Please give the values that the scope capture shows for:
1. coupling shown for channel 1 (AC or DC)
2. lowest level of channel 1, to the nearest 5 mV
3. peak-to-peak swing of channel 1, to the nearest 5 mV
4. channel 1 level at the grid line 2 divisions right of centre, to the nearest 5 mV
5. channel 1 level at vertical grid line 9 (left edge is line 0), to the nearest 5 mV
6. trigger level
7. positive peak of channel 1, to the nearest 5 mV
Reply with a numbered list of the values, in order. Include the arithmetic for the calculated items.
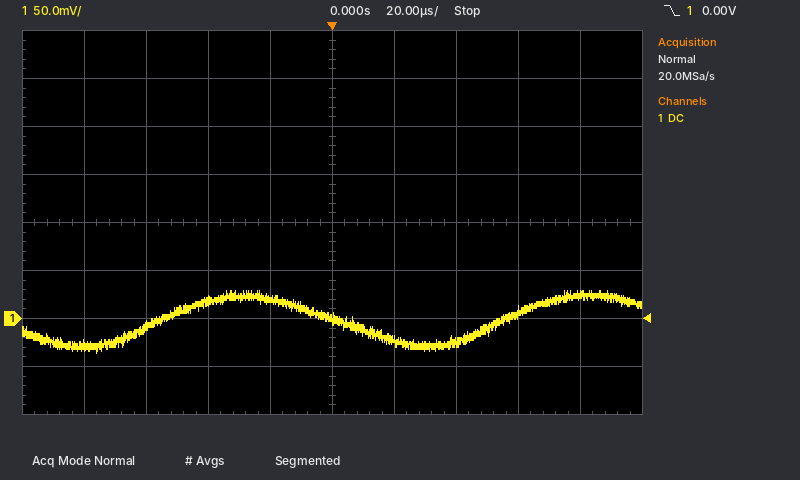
1. DC
2. -35 mV
3. 30 mV − (-35 mV) = 65 mV
4. -25 mV
5. 25 mV
6. 0.00 V
7. 30 mV
